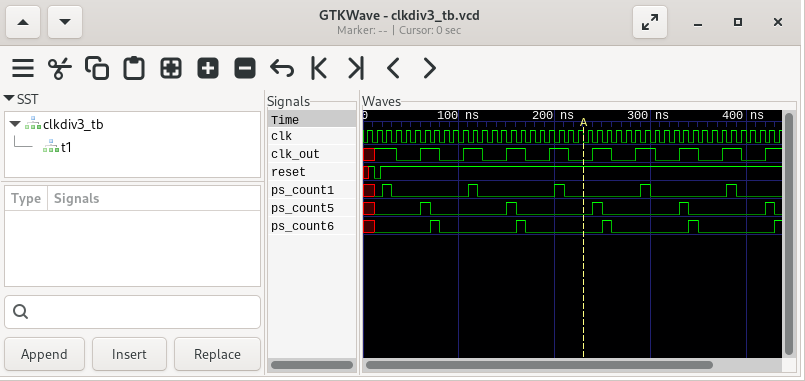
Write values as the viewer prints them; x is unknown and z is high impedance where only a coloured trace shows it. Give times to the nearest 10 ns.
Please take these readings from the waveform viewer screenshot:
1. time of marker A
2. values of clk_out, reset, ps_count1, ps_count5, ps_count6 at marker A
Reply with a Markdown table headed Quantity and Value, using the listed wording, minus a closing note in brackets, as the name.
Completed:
| Quantity | Value |
|---|---|
| time of marker A | 230 ns |
| values of clk_out, reset, ps_count1, ps_count5, ps_count6 at marker A | clk_out=0, reset=1, ps_count1=0, ps_count5=0, ps_count6=0 |
